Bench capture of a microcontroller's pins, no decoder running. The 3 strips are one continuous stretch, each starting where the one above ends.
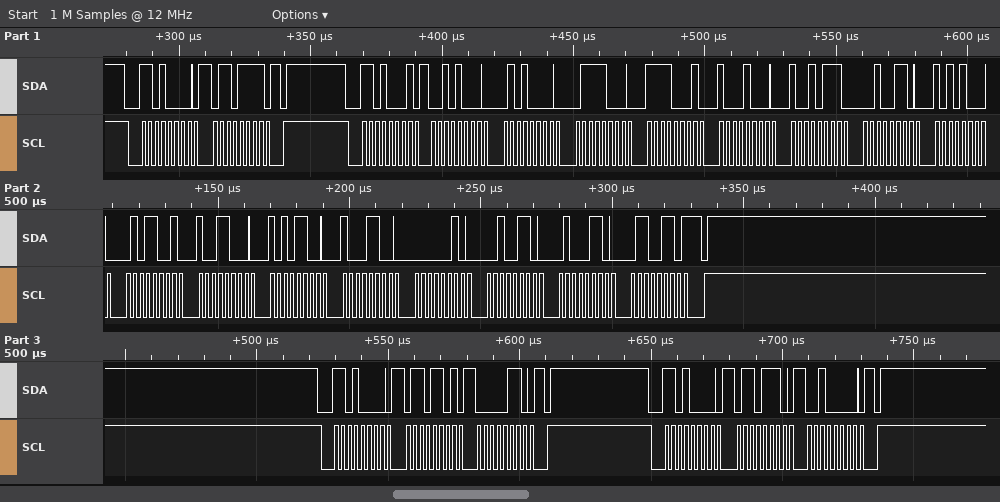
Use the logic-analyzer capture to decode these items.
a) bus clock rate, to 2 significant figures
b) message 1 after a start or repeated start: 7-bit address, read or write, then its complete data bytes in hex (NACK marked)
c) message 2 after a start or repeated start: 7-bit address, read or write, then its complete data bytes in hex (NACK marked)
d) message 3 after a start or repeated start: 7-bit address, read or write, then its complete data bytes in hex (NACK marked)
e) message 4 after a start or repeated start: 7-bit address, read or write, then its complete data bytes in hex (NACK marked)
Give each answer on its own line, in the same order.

400 kHz
0x68 write: 6F
0x68 read: 28 50 78 F1 88 97 26 A8 59 98 AC 8C 02 26 46 66 NACK
0x68 write: 6D 06
0x68 write: 6E 20
